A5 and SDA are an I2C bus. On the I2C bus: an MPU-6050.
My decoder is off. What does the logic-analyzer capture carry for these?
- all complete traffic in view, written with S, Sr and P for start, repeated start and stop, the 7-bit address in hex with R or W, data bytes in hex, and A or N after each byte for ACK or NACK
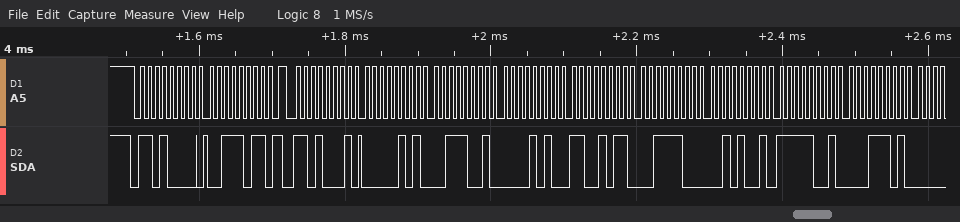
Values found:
S 68W A 3B A Sr 68R A 05 A 39 A 0A A CB A 3C A 29 A F9 A 1D A
